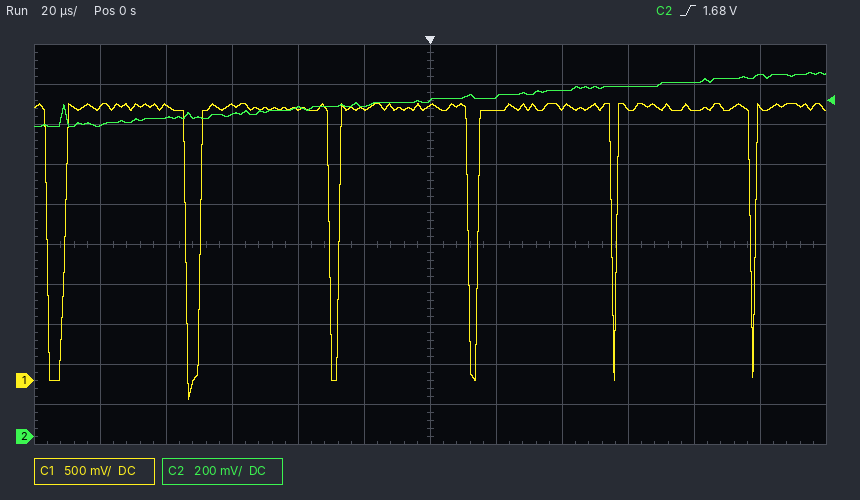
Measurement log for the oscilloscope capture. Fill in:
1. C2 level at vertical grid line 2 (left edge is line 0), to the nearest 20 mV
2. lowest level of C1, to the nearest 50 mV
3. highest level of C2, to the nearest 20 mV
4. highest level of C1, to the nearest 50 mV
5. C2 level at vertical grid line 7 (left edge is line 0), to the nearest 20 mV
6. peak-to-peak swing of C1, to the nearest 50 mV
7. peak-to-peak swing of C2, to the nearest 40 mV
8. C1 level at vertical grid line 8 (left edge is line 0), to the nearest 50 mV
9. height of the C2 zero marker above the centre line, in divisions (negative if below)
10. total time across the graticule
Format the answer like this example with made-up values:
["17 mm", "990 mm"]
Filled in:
["1.60 V", "-250 mV", "1.82 V", "3.45 V", "1.70 V", "3.70 V", "280 mV", "3.40 V", "-4.8 div", "240 µs"]
